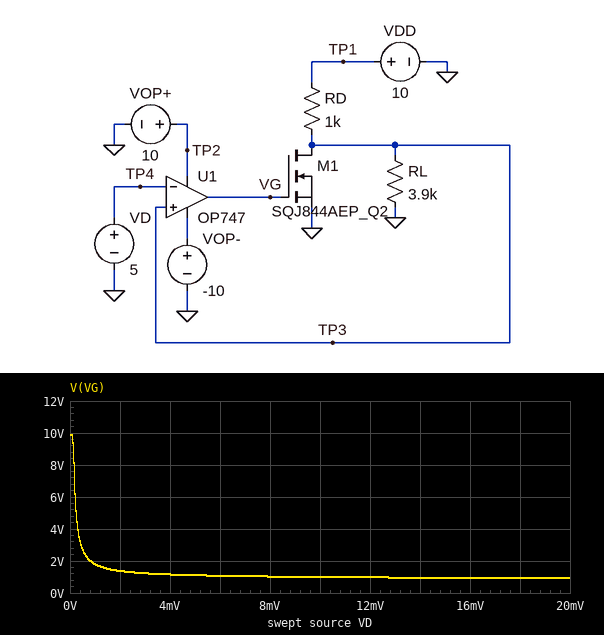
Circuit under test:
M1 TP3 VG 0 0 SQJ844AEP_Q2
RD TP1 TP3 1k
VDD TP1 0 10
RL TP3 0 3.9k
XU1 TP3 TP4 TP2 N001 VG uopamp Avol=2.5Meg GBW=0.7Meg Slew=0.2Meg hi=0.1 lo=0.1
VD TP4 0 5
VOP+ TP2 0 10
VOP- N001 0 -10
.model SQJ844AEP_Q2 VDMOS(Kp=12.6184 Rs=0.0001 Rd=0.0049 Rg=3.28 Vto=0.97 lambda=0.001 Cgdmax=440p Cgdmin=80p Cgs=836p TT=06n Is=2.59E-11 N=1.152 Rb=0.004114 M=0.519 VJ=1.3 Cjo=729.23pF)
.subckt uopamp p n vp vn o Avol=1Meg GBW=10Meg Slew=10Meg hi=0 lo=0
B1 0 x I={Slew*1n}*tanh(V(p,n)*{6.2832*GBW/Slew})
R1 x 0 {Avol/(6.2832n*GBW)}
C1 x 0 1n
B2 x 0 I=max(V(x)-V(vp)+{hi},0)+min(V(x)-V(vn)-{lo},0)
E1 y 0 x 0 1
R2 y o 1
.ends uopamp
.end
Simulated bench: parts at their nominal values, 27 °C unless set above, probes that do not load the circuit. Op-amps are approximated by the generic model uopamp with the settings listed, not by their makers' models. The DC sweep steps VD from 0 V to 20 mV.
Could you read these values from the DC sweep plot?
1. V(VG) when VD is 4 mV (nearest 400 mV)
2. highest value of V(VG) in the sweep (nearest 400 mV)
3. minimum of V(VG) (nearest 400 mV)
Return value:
1.2 V
10.0 V
800 mV
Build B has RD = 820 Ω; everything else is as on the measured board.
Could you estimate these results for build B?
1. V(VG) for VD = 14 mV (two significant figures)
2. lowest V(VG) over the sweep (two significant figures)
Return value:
980 mV
950 mV
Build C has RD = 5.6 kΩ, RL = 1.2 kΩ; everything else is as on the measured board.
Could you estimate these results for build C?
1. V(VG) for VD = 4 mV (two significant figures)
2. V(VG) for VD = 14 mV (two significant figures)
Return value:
890 mV
800 mV
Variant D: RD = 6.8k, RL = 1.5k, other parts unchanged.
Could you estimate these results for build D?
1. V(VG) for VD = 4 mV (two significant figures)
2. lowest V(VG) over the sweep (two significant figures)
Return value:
870 mV
790 mV
